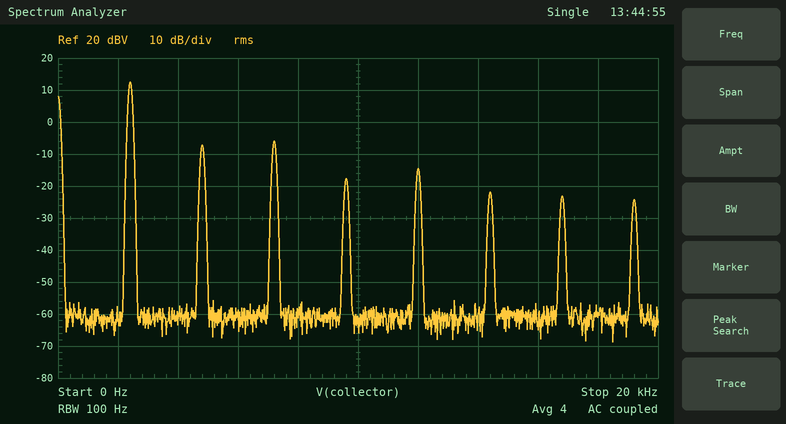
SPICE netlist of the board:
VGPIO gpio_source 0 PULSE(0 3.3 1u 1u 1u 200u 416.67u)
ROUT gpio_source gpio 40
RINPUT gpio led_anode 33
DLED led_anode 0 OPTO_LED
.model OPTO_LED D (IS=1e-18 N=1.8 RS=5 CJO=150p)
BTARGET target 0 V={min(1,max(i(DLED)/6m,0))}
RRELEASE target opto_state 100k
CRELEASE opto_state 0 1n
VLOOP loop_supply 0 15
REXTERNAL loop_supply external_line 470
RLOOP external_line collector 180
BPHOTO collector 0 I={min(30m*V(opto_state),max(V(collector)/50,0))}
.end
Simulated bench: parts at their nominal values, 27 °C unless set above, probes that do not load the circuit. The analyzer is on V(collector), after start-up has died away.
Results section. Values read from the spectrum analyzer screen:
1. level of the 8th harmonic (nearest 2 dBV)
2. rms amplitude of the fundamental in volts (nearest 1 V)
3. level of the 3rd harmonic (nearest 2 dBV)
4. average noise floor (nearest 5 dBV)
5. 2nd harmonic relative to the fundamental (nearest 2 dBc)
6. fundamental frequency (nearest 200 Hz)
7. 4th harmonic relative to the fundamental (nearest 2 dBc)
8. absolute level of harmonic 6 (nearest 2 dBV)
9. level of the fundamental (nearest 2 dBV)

-24 dBV
4 V
-6 dBV
-60 dBV
-20 dBc
2.4 kHz
-30 dBc
-22 dBV
12 dBV
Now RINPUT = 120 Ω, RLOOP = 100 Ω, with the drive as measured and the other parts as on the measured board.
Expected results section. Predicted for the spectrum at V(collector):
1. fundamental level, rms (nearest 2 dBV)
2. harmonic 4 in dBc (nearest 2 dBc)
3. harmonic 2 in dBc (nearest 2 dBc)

12 dBV
-36 dBc
-28 dBc
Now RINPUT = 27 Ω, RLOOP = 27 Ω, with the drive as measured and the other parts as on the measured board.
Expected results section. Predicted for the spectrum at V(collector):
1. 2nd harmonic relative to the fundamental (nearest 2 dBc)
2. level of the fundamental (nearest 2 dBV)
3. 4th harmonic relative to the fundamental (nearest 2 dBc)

-30 dBc
12 dBV
-36 dBc
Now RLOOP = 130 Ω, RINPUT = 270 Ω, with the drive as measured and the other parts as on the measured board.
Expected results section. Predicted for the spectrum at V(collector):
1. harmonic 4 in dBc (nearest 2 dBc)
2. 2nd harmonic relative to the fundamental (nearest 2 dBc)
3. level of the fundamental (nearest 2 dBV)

-36 dBc
-30 dBc
12 dBV
